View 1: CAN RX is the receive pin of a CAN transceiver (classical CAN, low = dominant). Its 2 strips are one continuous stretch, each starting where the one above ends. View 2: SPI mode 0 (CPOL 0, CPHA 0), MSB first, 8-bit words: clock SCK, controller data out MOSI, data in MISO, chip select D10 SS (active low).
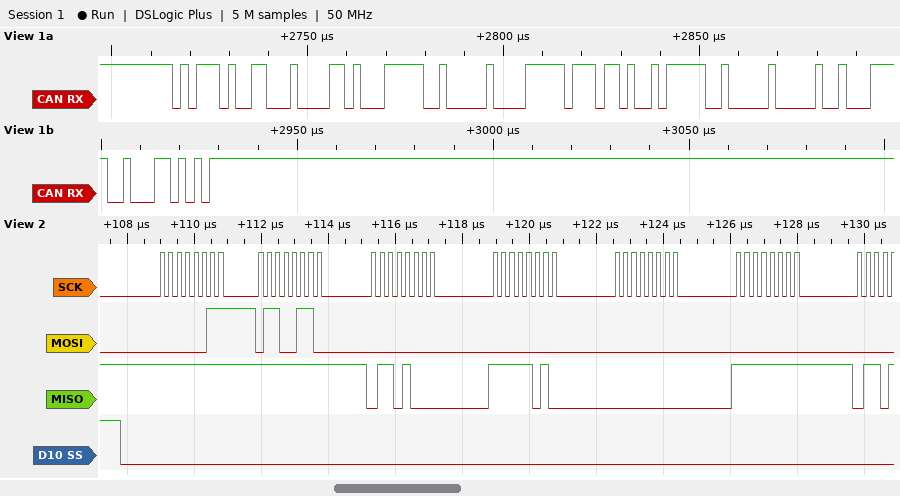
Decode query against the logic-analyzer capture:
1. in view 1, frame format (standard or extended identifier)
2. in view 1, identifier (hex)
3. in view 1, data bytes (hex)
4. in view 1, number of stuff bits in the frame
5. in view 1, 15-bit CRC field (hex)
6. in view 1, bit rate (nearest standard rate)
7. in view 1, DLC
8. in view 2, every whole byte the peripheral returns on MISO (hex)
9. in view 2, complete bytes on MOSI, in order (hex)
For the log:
standard
0x5D3
68 FA 00 FF 69 7D 00 08
6
0x791A
500 kbit/s
8
FF FF 68 FA 00 FF
03 66 00 00 00 00
